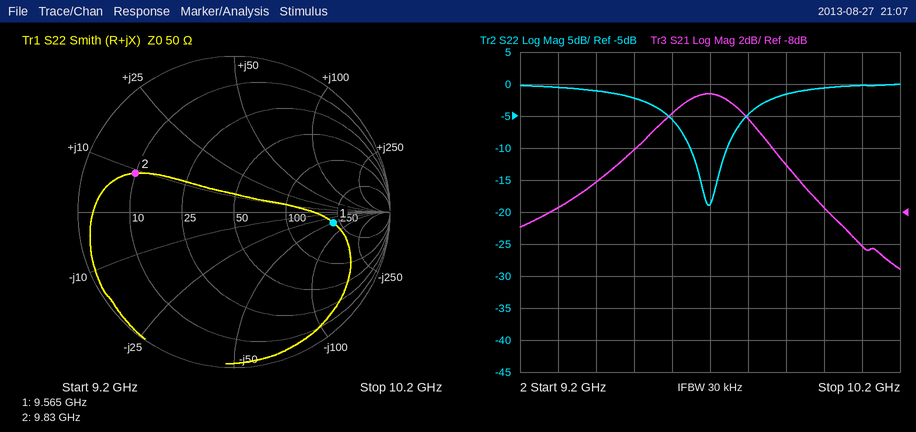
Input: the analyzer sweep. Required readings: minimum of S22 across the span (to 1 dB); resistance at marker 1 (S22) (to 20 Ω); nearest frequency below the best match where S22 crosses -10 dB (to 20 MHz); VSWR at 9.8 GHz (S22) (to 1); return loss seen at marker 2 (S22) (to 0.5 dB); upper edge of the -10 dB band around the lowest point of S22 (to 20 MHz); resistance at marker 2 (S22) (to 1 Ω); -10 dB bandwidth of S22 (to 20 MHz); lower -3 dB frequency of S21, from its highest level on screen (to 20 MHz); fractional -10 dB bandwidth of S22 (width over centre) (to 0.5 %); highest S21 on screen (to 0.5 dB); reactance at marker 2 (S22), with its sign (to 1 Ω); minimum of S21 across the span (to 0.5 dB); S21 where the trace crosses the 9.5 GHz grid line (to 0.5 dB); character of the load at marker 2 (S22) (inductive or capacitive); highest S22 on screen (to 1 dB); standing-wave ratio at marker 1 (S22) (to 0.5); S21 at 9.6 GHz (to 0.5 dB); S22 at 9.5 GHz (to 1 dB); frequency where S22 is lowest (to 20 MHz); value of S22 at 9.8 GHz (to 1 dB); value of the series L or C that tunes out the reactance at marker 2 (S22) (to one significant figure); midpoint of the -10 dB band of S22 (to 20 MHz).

-19 dB
220 Ω
9.64 GHz
4
3.5 dB
9.74 GHz
10 Ω
100 MHz
9.52 GHz
1.0 %
-0.5 dB
+9 Ω
-11.5 dB
-4.0 dB
inductive
0 dB
4.5
-2.0 dB
-2 dB
9.70 GHz
-5 dB
2 pF
9.70 GHz
